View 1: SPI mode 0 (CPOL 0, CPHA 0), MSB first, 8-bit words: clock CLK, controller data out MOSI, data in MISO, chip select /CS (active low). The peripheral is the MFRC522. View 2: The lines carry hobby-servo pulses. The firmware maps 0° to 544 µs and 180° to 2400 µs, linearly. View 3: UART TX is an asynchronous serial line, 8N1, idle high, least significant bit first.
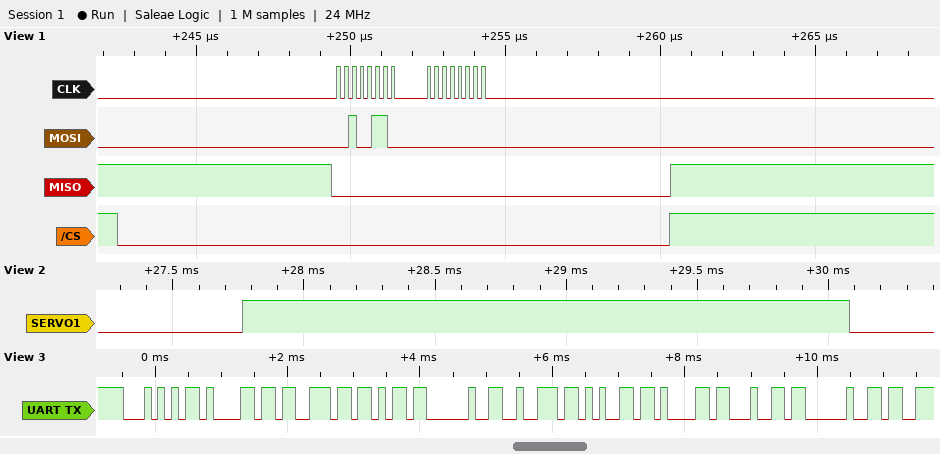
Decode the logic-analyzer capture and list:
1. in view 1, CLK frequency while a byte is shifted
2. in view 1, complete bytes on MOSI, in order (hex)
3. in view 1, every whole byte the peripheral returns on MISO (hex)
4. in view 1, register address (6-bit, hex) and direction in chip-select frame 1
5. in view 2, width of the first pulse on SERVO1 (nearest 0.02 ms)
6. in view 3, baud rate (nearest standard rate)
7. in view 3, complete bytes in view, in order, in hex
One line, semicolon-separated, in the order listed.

4 MHz; 26 00; 00 00; 0x13 write; 2.32 ms; 9600 baud; 0x54 0x61 0x73 0x6B 0x20 0x72 0x65 0x61 0x64 0x20
